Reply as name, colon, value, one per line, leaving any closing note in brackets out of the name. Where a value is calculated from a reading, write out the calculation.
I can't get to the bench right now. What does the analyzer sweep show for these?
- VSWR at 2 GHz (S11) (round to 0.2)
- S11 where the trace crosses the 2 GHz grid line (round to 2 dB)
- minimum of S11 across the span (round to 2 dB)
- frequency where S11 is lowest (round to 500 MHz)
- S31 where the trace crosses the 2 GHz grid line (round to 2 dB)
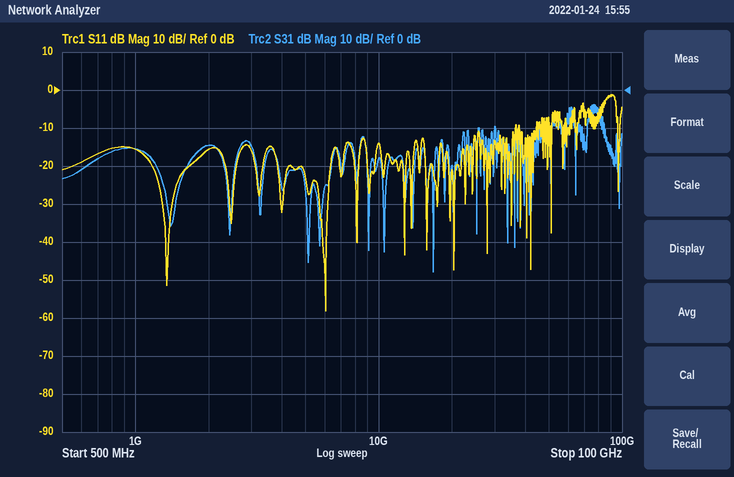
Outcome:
VSWR at 2 GHz (S11): |Γ| = 10^(-16/20) = 0.1585; VSWR = (1 + 0.1585)/(1 − 0.1585) ≈ 1.4
S11 where the trace crosses the 2 GHz grid line: -16 dB
minimum of S11 across the span: -58 dB
frequency where S11 is lowest: 6.0 GHz
S31 where the trace crosses the 2 GHz grid line: -14 dB
